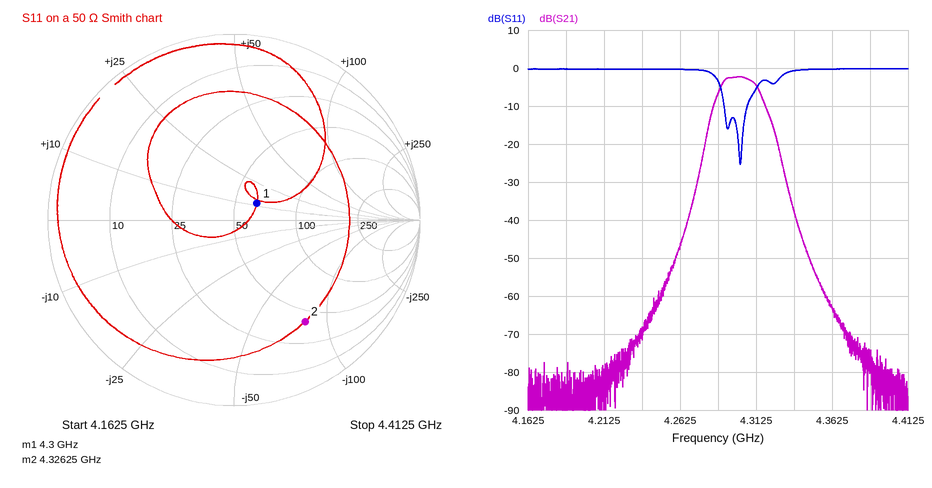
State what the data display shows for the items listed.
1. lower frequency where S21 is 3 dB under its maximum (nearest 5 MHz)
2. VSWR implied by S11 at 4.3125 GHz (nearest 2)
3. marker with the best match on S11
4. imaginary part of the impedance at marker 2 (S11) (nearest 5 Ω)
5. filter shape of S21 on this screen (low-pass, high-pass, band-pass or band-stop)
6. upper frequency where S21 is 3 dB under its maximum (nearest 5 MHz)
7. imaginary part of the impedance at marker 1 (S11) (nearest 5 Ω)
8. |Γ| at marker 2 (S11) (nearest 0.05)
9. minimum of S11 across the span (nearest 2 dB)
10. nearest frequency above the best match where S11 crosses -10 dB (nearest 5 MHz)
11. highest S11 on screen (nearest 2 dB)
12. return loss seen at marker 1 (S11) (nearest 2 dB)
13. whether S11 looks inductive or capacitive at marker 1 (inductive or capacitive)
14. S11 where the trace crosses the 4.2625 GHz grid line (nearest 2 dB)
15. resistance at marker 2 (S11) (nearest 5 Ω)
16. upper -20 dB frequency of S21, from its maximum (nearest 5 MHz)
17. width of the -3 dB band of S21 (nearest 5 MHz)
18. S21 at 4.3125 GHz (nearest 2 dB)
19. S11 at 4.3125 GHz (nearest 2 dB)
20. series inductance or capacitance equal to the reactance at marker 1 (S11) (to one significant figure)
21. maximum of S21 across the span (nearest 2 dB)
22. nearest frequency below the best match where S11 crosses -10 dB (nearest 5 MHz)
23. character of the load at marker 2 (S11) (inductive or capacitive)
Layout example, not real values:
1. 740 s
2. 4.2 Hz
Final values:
1. 4.290 GHz
2. 4
3. marker 1
4. -80 Ω
5. band-pass
6. 4.315 GHz
7. +10 Ω
8. 0.65
9. -26 dB
10. 4.305 GHz
11. 0 dB
12. 16 dB
13. inductive
14. 0 dB
15. 40 Ω
16. 4.330 GHz
17. 25 MHz
18. -4 dB
19. -6 dB
20. 400 pH
21. -2 dB
22. 4.290 GHz
23. capacitive
